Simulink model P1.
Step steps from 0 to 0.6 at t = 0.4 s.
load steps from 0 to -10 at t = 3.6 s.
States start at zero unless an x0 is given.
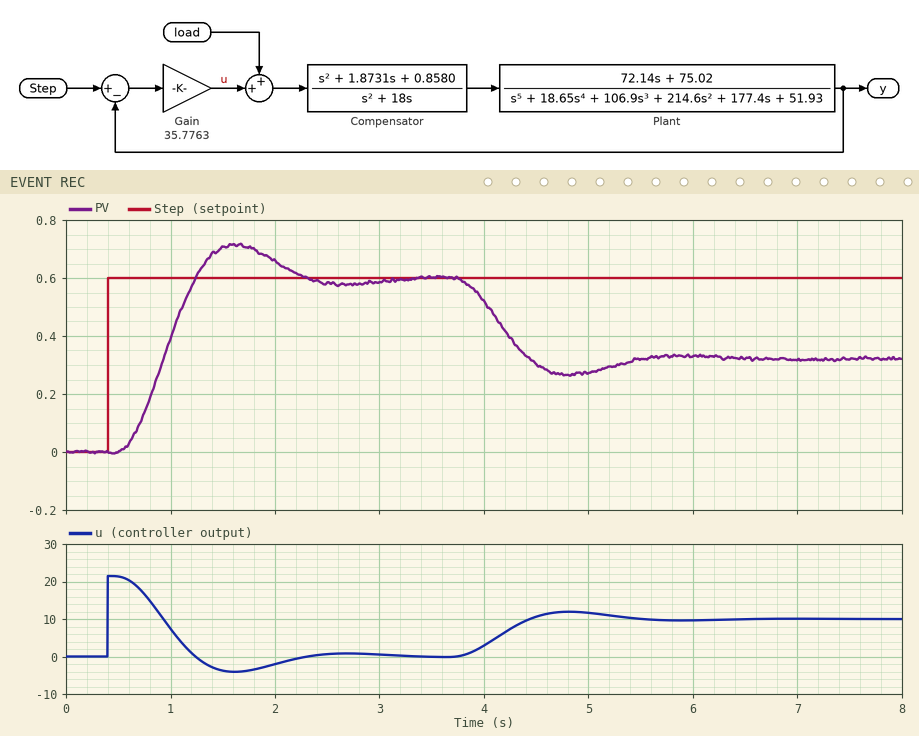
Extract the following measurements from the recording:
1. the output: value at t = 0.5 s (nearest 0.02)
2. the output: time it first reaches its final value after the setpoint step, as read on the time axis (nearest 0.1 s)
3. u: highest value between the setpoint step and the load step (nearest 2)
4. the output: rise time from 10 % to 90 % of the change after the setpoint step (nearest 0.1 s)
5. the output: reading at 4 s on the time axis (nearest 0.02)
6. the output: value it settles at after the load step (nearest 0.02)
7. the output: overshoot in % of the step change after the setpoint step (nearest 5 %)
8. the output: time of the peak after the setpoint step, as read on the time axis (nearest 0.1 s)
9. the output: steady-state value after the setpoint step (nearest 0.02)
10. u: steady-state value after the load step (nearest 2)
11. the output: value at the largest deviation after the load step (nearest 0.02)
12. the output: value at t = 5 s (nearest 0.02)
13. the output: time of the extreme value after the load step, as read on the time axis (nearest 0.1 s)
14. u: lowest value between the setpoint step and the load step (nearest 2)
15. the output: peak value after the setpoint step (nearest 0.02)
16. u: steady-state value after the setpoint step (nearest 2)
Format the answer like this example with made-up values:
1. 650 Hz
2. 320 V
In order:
1. 0.00
2. 1.2 s
3. 22
4. 0.5 s
5. 0.52
6. 0.32
7. 20 %
8. 1.6 s
9. 0.60
10. 10
11. 0.26
12. 0.28
13. 4.8 s
14. -4
15. 0.72
16. 0
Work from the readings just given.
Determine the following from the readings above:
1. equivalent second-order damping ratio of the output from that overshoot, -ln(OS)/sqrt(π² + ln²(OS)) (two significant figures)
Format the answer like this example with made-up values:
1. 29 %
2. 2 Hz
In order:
1. 0.46
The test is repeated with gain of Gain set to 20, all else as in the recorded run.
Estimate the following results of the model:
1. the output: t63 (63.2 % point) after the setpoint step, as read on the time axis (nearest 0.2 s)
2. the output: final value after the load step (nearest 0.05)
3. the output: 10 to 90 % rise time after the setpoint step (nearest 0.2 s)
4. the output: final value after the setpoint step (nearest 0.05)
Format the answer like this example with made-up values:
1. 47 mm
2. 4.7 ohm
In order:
1. 1.2 s
2. 0.10
3. 1.0 s
4. 0.60
